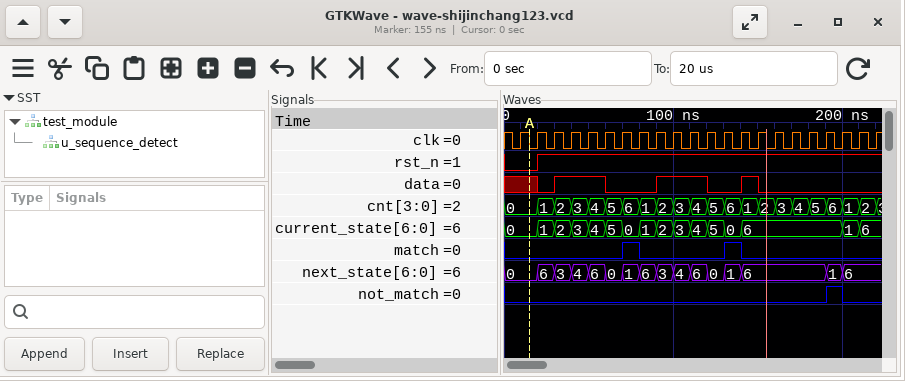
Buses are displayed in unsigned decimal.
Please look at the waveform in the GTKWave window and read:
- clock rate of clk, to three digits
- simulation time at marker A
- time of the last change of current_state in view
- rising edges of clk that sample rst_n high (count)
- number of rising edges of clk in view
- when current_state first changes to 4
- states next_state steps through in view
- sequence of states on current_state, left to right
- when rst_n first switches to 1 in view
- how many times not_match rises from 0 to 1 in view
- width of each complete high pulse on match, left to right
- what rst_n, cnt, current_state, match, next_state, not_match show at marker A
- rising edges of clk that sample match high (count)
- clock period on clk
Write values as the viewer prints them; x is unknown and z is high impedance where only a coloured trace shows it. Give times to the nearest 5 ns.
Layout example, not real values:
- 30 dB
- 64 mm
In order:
- 100 MHz
- 15 ns
- 210 ns
- 20
- 22
- 50 ns
- 0, 6, 3, 4, 6, 0, 1, 6, 3, 4, 6, 0, 1, 6, 1, 6
- 0, 1, 2, 3, 4, 5, 0, 1, 2, 3, 4, 5, 0, 6, 1, 6
- 20 ns
- 1
- 10 ns, 10 ns
- rst_n=0, cnt=0, current_state=0, match=0, next_state=0, not_match=0
- 2
- 10 ns
